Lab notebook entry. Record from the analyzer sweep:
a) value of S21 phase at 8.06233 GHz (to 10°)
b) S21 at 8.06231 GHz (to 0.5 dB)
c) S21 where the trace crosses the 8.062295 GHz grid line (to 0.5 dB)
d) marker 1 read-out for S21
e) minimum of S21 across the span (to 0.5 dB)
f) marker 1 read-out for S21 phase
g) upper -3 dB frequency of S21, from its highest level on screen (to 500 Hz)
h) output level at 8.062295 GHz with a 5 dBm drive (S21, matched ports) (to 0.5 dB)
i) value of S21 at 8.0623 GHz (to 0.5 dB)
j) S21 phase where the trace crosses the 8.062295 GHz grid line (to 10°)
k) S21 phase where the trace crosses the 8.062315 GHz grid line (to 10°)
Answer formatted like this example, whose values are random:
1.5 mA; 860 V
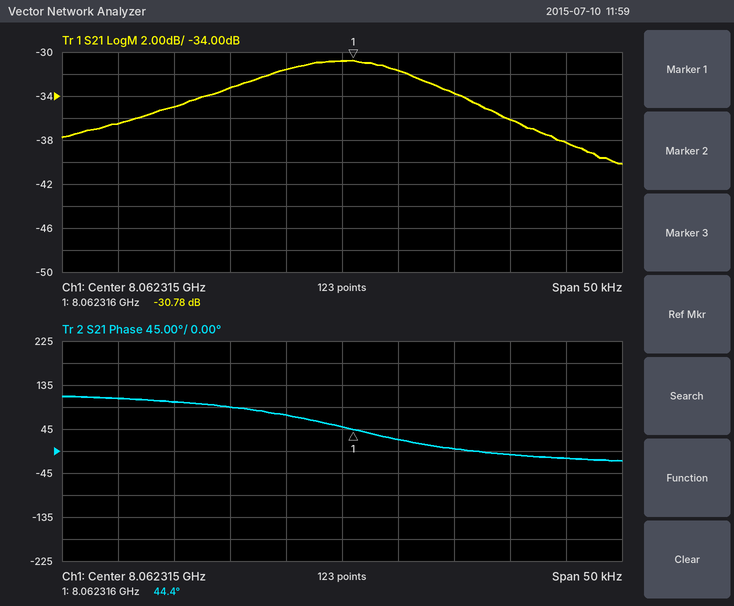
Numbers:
-10°; -31.5 dB; -36.5 dB; -30.78 dB; -40.0 dB; 44.4°; 8.0623250 GHz; -31.5 dBm; -35.0 dB; 110°; 50°
